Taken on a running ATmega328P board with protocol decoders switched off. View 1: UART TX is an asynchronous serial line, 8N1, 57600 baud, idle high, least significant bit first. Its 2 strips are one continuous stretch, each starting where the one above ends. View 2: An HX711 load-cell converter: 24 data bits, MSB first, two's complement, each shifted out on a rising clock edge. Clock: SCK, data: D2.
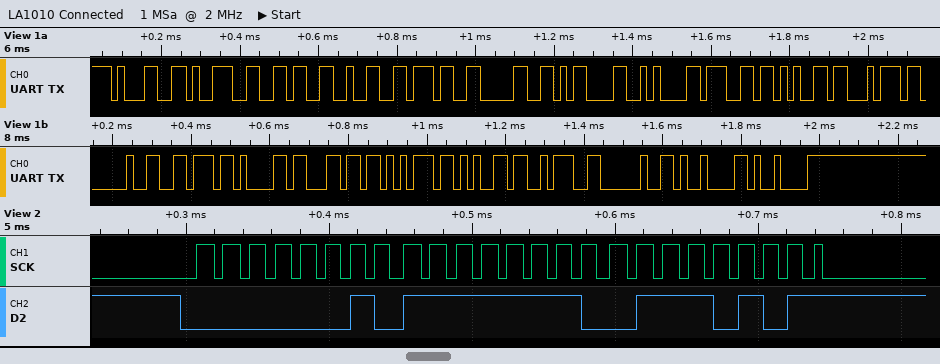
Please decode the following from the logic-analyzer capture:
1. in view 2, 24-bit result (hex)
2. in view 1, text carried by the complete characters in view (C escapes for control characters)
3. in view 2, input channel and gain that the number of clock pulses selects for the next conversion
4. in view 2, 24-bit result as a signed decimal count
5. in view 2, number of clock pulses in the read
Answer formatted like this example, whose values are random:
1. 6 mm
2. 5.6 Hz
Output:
1. 0x02FE75
2. "196270\r\nget value: \t\t"
3. channel A, gain 128
4. 196213
5. 25
